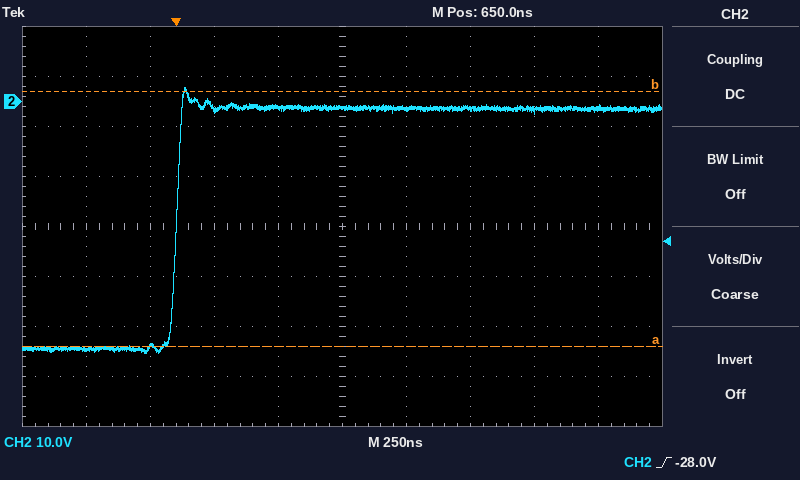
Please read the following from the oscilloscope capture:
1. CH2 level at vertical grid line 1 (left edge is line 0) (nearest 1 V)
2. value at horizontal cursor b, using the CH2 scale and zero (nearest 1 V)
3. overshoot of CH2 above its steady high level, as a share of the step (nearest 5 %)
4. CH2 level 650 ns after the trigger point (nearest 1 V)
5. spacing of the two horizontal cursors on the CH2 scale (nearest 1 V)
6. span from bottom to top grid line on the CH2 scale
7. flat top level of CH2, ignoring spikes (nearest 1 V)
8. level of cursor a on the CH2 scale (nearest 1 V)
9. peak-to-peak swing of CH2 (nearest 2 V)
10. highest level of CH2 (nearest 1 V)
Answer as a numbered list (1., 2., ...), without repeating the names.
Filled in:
1. -50 V
2. 2 V
3. 10 %
4. -1 V
5. 51 V
6. 80 V
7. -1 V
8. -49 V
9. 54 V
10. 3 V
